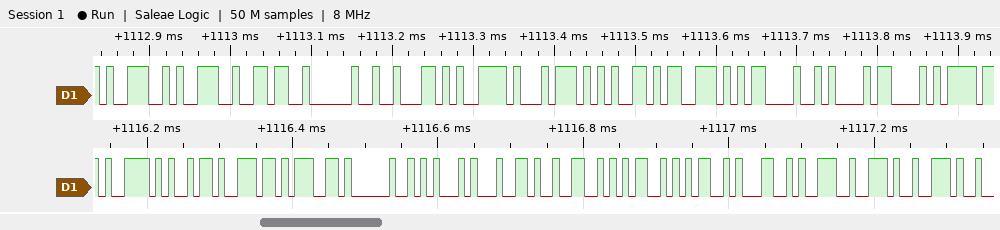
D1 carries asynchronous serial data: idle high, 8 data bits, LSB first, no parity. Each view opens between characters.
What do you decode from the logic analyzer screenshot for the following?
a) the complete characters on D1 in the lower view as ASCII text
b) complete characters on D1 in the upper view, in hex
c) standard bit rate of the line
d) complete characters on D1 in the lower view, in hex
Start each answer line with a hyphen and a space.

- "ying Ed25519.."
- 39, 39, 36, 20, 62, 79, 74, 65, 73, 0D, 0A, 43
- 115200 baud
- 79, 69, 6E, 67, 20, 45, 64, 32, 35, 35, 31, 39, 2E, 2E
